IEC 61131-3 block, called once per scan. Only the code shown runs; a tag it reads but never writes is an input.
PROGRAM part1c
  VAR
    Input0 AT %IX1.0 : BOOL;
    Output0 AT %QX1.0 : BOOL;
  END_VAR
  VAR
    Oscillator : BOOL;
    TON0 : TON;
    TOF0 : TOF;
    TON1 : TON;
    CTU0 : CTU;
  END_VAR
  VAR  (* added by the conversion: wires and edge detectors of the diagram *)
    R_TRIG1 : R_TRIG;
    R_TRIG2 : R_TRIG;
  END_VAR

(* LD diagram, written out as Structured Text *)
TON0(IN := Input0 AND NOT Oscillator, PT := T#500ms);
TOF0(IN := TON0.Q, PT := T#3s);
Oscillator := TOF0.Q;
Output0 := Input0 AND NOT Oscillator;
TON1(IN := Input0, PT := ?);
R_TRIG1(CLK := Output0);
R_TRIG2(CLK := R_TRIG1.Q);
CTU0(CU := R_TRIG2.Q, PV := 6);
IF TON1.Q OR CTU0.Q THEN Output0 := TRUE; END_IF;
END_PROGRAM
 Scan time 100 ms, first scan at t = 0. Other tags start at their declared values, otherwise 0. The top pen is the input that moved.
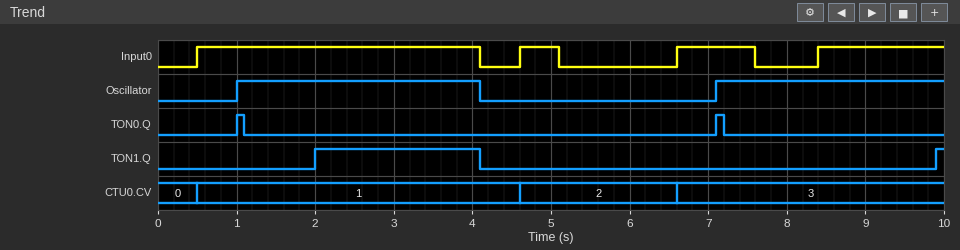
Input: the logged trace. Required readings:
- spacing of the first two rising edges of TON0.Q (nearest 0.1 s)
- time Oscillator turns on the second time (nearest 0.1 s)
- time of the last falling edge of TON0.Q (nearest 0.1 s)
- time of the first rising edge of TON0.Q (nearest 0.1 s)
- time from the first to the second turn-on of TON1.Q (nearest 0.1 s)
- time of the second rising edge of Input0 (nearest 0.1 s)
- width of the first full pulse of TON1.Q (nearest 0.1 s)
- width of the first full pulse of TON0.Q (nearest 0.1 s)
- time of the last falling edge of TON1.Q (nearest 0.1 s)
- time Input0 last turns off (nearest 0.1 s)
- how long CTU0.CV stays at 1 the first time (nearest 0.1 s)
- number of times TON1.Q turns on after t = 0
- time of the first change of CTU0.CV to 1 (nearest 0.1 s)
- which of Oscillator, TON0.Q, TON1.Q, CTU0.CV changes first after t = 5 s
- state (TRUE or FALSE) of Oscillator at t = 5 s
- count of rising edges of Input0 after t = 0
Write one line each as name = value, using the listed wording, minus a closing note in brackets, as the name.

spacing of the first two rising edges of TON0.Q = 6.1 s
time Oscillator turns on the second time = 7.1 s
time of the last falling edge of TON0.Q = 7.2 s
time of the first rising edge of TON0.Q = 1.0 s
time from the first to the second turn-on of TON1.Q = 7.9 s
time of the second rising edge of Input0 = 4.6 s
width of the first full pulse of TON1.Q = 2.1 s
width of the first full pulse of TON0.Q = 0.1 s
time of the last falling edge of TON1.Q = 4.1 s
time Input0 last turns off = 7.6 s
how long CTU0.CV stays at 1 the first time = 4.1 s
number of times TON1.Q turns on after t = 0 = 2
time of the first change of CTU0.CV to 1 = 0.5 s
which of Oscillator, TON0.Q, TON1.Q, CTU0.CV changes first after t = 5 s = CTU0.CV
state (TRUE or FALSE) of Oscillator at t = 5 s = FALSE
count of rising edges of Input0 after t = 0 = 4
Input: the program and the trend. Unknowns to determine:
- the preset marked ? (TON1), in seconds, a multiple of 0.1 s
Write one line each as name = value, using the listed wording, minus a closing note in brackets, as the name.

the preset marked ? (TON1), in seconds, a multiple of 0.1 s = 1.5 s
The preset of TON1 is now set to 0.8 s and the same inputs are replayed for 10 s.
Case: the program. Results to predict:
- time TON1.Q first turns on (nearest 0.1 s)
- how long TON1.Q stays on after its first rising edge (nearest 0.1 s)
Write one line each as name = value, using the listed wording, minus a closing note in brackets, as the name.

time TON1.Q first turns on = 1.3 s
how long TON1.Q stays on after its first rising edge = 2.8 s
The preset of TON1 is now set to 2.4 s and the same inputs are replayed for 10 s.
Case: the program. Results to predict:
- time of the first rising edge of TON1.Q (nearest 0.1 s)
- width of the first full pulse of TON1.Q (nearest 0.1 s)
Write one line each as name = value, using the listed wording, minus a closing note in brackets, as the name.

time of the first rising edge of TON1.Q = 2.9 s
width of the first full pulse of TON1.Q = 1.2 s
